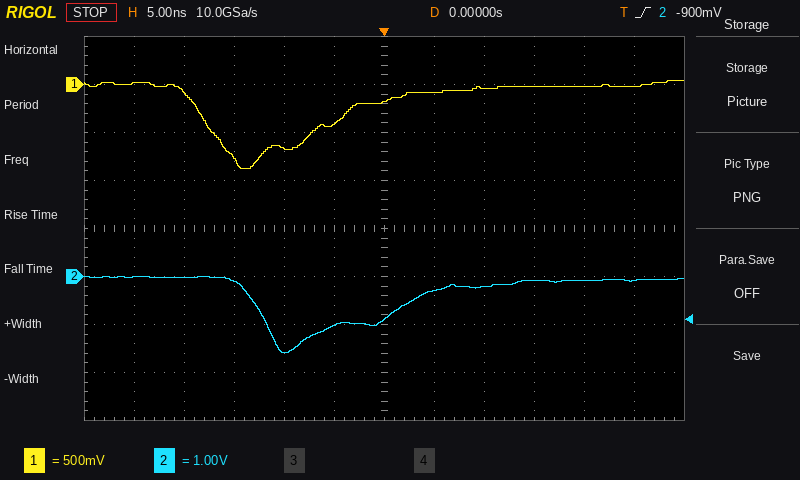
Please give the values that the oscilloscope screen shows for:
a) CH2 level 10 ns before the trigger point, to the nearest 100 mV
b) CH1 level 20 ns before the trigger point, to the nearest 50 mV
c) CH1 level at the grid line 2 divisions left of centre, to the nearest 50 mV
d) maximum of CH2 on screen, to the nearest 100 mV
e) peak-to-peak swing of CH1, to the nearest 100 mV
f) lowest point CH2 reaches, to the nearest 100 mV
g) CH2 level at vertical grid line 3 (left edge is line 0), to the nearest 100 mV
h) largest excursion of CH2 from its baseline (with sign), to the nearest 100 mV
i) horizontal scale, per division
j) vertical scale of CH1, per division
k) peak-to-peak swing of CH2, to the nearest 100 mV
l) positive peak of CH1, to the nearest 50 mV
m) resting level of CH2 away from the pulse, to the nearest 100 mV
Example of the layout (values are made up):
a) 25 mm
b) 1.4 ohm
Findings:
a) -1.6 V
b) -100 mV
c) -650 mV
d) 0.0 V
e) 900 mV
f) -1.6 V
g) -100 mV
h) -1.5 V
i) 5 ns
j) 500 mV
k) 1.6 V
l) 50 mV
m) -100 mV
